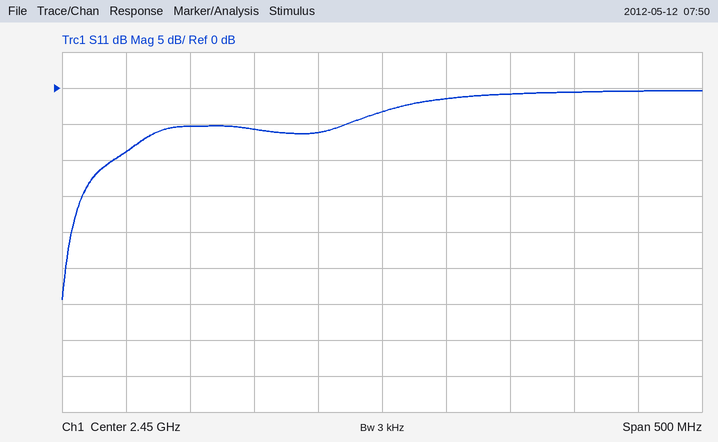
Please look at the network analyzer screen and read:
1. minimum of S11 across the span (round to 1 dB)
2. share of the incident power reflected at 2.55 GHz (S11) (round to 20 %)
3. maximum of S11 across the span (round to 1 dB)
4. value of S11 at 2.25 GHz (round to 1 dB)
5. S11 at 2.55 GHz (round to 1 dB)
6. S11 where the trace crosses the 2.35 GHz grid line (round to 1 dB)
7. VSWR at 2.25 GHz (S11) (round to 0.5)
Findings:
-29 dB
80 %
0 dB
-9 dB
-1 dB
-6 dB
2.0
